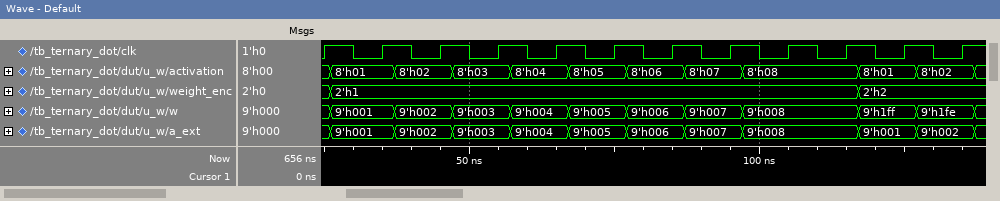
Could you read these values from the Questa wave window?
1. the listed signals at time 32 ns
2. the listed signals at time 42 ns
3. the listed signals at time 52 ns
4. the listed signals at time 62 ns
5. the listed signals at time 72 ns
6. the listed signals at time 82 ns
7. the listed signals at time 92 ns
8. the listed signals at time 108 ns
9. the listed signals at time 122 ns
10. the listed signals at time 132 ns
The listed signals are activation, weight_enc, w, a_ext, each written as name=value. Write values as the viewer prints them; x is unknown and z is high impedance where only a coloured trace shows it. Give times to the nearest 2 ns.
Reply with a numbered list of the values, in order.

1. activation=8'h01, weight_enc=2'h1, w=9'h001, a_ext=9'h001
2. activation=8'h02, weight_enc=2'h1, w=9'h002, a_ext=9'h002
3. activation=8'h03, weight_enc=2'h1, w=9'h003, a_ext=9'h003
4. activation=8'h04, weight_enc=2'h1, w=9'h004, a_ext=9'h004
5. activation=8'h05, weight_enc=2'h1, w=9'h005, a_ext=9'h005
6. activation=8'h06, weight_enc=2'h1, w=9'h006, a_ext=9'h006
7. activation=8'h07, weight_enc=2'h1, w=9'h007, a_ext=9'h007
8. activation=8'h08, weight_enc=2'h1, w=9'h008, a_ext=9'h008
9. activation=8'h01, weight_enc=2'h2, w=9'h1ff, a_ext=9'h001
10. activation=8'h02, weight_enc=2'h2, w=9'h1fe, a_ext=9'h002
